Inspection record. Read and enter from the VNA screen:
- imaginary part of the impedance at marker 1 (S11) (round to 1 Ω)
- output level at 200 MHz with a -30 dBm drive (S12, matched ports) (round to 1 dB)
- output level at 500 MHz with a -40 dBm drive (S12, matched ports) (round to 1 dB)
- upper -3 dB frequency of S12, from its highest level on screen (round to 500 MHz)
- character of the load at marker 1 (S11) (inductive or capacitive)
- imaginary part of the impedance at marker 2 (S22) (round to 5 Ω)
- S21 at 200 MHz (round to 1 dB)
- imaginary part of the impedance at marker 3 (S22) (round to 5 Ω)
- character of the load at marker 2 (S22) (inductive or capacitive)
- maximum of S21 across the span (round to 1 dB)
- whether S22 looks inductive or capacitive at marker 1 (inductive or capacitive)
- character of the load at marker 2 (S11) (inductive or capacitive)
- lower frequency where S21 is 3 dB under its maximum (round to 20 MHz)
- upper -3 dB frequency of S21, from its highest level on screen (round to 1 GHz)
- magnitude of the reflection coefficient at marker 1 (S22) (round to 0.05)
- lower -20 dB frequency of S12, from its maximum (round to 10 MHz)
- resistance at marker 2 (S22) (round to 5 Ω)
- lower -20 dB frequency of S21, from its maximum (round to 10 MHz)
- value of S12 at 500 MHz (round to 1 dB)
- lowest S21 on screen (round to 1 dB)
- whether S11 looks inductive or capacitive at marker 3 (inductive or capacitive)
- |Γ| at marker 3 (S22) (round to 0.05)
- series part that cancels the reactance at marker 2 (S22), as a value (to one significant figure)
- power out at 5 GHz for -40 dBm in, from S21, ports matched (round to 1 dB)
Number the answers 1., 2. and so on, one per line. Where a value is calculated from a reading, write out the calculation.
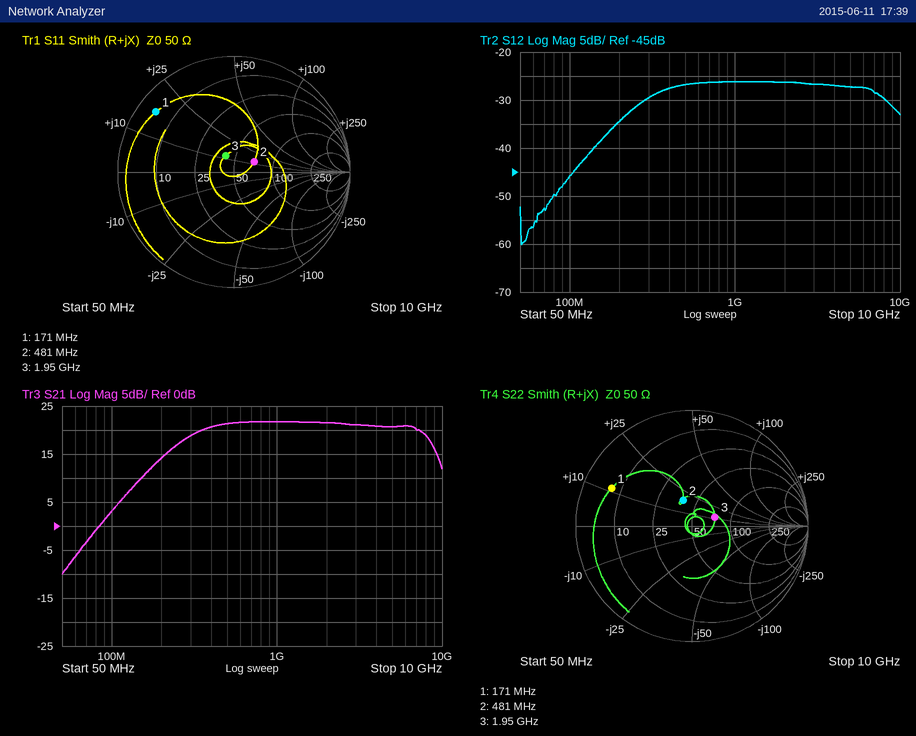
1. +17 Ω
2. -30 dBm + (-34 dB) = -64 dBm
3. -40 dBm + (-27 dB) = -67 dBm
4. 7.5 GHz
5. inductive
6. +20 Ω
7. 14 dB
8. +10 Ω
9. inductive
10. 22 dB
11. inductive
12. inductive
13. 300 MHz
14. 8 GHz
15. 0.75
16. 100 MHz
17. 40 Ω
18. 90 MHz
19. -27 dB
20. -10 dB
21. inductive
22. 0.20
23. C = 1/(2π × 481 MHz × 20 Ω) ≈ 16.5 pF, so 20 pF to one significant figure
24. -40 dBm + (21 dB) = -19 dBm
